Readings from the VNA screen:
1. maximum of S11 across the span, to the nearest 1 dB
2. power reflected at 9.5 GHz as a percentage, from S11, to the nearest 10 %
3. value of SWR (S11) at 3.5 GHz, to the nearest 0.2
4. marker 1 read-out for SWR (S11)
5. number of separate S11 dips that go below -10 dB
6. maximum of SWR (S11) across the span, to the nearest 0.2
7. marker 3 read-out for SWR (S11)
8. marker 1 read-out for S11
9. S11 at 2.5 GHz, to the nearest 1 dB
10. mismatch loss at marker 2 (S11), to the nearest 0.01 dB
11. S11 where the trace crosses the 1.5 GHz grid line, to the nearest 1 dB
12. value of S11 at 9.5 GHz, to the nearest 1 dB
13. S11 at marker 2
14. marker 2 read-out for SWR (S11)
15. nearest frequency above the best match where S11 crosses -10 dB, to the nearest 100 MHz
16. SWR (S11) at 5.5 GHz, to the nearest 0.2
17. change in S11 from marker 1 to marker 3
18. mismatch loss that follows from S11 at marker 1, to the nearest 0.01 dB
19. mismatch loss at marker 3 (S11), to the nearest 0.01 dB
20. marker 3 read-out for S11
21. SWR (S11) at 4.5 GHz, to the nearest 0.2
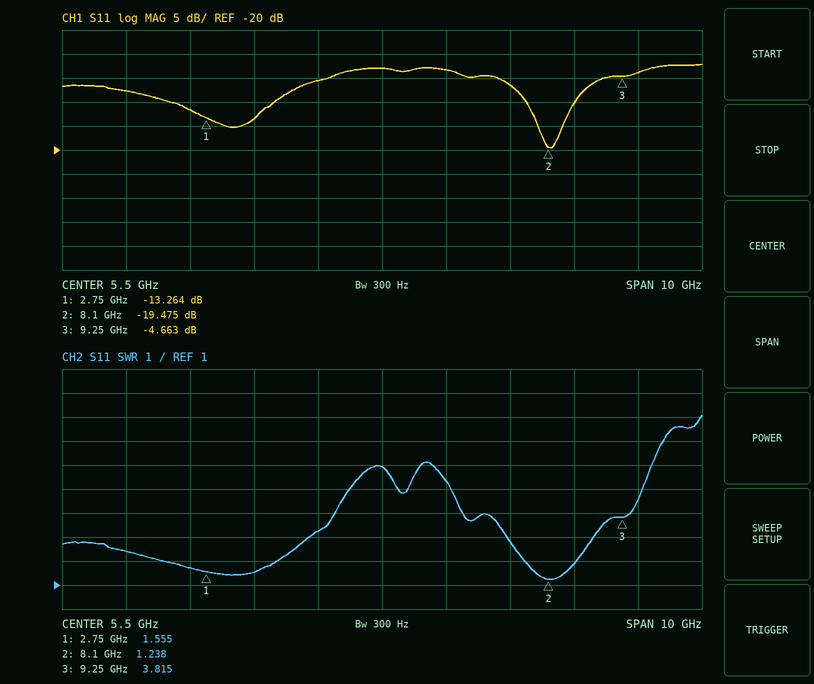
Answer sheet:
-2 dB
40 %
1.6
1.555
2
8.0
3.815
-13.264 dB
-12 dB
0.05 dB
-8 dB
-4 dB
-19.475 dB
1.238
8.5 GHz
6.0
8.601 dB
0.21 dB
1.82 dB
-4.663 dB
3.2
